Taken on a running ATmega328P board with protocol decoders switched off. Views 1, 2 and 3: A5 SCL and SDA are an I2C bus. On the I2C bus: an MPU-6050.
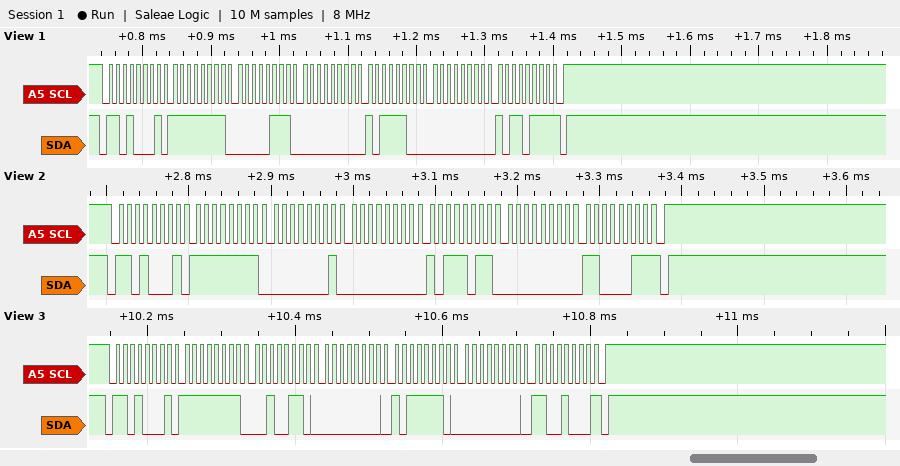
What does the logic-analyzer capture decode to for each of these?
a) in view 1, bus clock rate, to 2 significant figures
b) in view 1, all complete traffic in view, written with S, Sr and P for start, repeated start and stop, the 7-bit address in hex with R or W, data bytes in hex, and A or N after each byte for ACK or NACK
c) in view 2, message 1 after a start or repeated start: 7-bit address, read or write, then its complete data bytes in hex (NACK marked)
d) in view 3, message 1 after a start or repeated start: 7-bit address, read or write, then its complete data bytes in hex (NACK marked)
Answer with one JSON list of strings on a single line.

["100 kHz", "S 68R A FF A 07 A 00 A BC A 00 A B7 N P", "0x68 read: FF 01 00 BB 00 C3 NACK", "0x68 read: FF 26 00 BE 00 C8 NACK"]
